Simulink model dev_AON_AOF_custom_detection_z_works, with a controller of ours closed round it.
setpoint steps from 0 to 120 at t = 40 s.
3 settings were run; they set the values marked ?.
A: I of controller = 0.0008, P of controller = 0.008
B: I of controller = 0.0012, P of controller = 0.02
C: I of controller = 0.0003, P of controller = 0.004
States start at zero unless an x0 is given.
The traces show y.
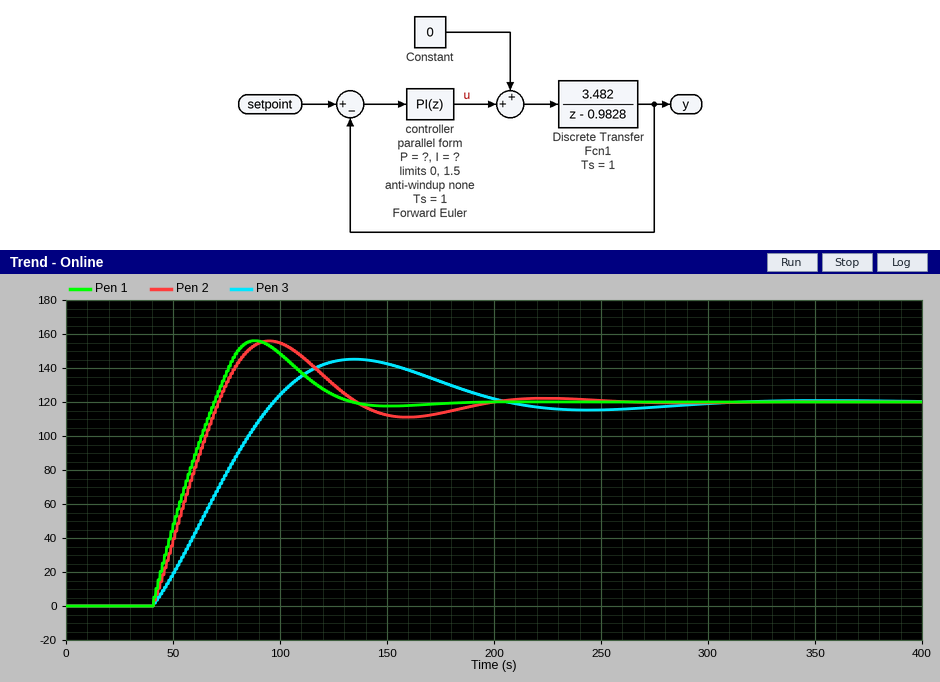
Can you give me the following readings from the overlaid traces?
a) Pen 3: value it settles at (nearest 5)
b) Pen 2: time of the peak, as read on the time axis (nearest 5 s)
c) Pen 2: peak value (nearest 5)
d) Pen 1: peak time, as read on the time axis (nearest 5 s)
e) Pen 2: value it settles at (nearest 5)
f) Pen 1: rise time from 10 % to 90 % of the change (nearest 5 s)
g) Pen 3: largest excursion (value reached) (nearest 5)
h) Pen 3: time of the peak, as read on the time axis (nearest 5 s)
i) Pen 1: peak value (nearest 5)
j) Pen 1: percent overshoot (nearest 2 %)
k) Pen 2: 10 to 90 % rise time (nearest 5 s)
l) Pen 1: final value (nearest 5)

120
95 s
155
90 s
120
25 s
145
135 s
155
30 %
25 s
120
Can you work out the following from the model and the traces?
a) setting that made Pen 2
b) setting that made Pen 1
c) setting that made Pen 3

A
B
C
